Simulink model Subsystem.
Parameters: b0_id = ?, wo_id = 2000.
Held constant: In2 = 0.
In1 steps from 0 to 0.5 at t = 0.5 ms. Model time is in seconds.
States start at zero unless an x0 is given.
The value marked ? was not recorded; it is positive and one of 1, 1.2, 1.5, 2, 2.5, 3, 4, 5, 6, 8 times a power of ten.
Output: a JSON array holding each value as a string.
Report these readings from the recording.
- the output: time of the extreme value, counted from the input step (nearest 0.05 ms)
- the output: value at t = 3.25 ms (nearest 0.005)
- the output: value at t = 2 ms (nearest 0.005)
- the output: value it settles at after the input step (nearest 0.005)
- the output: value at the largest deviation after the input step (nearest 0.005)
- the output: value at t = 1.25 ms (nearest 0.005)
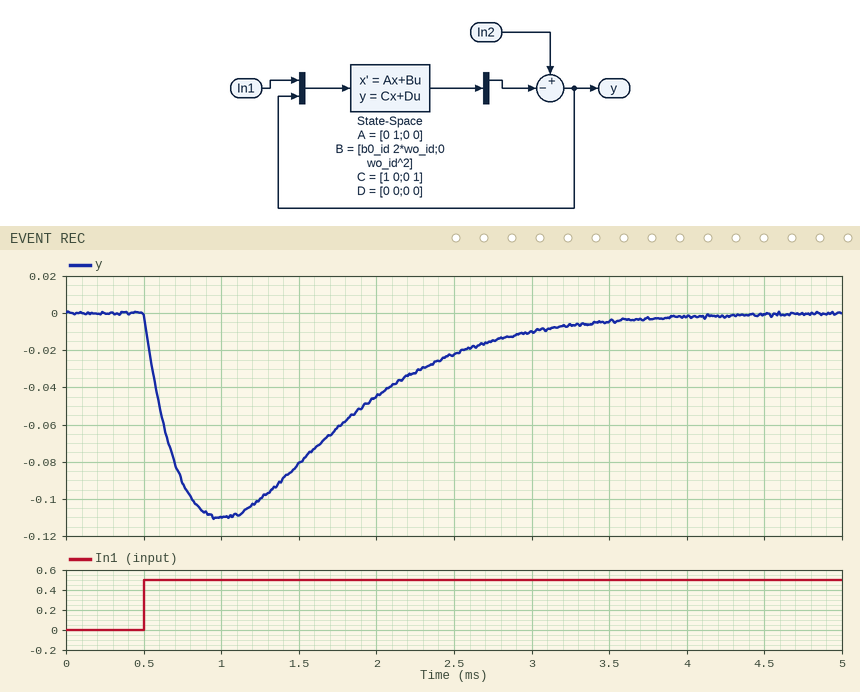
["0.50 ms", "-0.005", "-0.045", "0.000", "-0.110", "-0.100"]
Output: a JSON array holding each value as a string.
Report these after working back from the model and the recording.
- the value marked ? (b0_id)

["1200"]
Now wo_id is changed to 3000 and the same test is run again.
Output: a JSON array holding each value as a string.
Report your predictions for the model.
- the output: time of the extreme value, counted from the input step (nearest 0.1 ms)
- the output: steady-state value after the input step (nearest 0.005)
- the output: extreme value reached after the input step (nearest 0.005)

["0.3 ms", "0.000", "-0.075"]
